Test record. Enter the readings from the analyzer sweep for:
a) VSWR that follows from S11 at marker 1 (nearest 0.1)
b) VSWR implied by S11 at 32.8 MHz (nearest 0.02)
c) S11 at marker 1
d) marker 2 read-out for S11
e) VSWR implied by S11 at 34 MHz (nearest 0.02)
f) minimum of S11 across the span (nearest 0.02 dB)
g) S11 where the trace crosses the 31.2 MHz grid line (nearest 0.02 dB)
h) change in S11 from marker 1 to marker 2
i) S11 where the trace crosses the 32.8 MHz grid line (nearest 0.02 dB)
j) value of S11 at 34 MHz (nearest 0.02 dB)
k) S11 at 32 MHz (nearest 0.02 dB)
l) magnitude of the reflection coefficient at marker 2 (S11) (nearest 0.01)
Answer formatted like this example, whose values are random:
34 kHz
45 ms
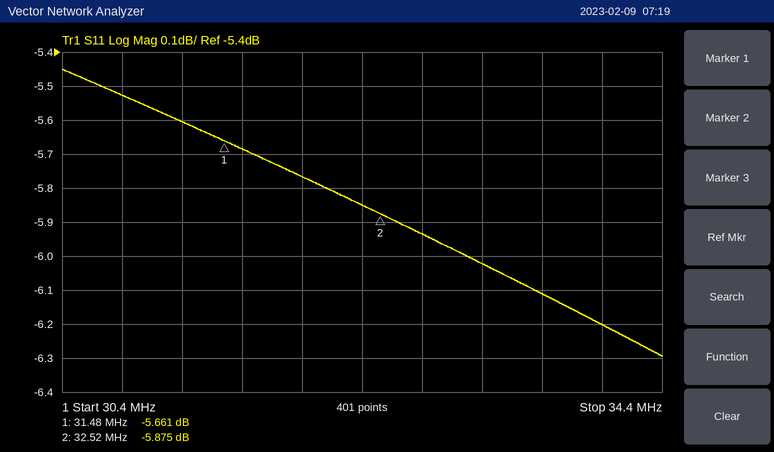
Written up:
3.2
3.04
-5.661 dB
-5.875 dB
2.92
-6.30 dB
-5.60 dB
-0.214 dB
-5.94 dB
-6.20 dB
-5.76 dB
0.51
